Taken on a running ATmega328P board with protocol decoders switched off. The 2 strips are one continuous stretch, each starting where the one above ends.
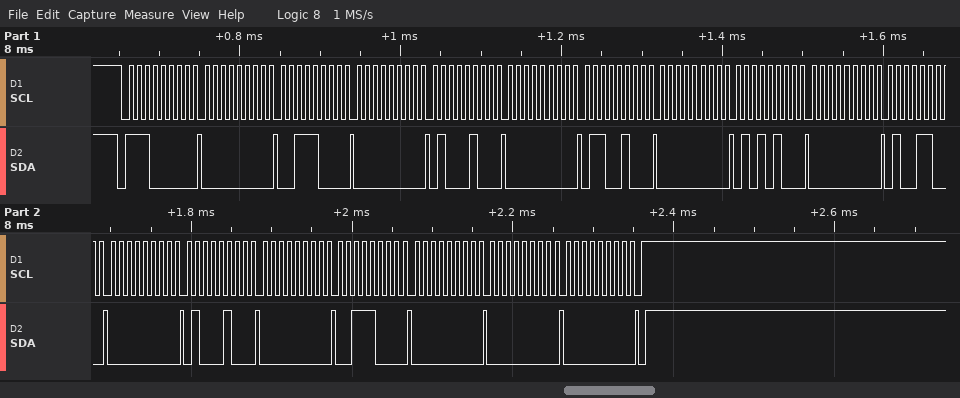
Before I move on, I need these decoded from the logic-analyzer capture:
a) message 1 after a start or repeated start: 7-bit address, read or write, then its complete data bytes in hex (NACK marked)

0x70 write: 00 38 00 44 00 64 00 54 00 4C 00 44 00 38 00 00 00
